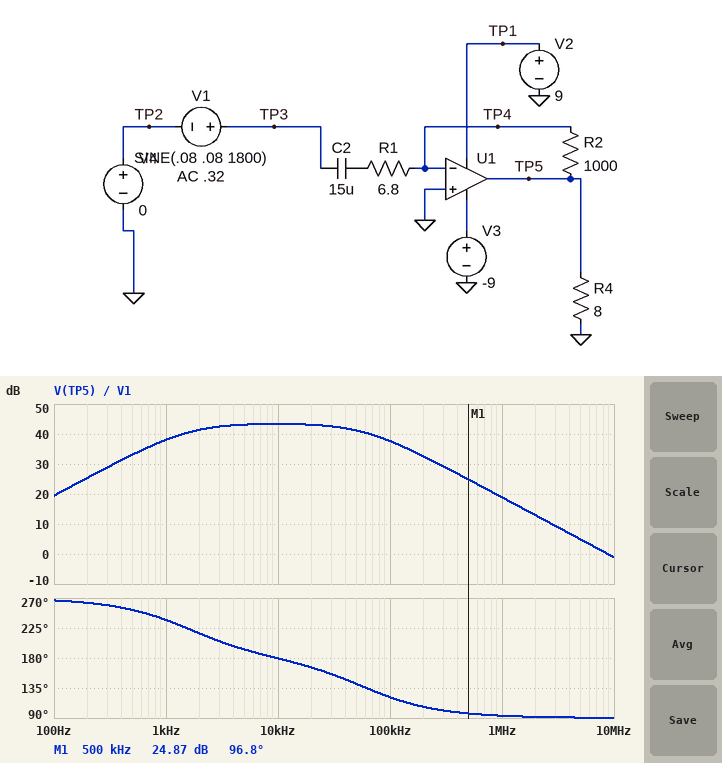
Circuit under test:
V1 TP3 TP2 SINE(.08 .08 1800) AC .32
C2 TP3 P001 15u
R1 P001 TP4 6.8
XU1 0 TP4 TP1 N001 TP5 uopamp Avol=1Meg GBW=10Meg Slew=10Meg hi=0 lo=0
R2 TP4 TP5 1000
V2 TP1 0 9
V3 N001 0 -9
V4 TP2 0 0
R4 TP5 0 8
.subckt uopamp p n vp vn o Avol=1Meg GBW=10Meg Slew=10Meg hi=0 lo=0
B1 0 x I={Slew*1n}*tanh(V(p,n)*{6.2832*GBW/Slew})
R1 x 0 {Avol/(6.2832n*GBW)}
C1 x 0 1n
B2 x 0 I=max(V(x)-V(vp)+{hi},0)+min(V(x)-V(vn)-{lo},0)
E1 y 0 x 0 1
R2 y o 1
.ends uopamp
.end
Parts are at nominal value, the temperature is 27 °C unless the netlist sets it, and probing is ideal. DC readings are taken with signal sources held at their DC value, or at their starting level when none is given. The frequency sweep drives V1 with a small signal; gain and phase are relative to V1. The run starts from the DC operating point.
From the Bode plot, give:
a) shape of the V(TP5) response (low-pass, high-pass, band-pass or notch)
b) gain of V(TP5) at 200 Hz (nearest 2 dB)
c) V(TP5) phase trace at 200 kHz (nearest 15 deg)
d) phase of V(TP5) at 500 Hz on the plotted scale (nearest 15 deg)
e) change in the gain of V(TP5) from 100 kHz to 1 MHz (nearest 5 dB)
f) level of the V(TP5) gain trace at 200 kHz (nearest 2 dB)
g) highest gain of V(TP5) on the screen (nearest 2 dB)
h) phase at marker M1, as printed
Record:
band-pass
26 dB
105 deg
255 deg
-20 dB
32 dB
44 dB
96.8 deg
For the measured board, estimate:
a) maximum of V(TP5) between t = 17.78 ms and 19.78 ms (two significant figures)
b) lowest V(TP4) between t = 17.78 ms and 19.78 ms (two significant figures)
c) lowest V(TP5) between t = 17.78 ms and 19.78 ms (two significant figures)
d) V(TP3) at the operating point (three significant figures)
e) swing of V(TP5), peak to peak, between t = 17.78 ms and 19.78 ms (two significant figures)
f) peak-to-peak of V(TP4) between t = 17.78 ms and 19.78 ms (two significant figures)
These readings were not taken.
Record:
8.0 V
-8.5 mV
-8.0 V
80.0 mV
16 V
17 mV
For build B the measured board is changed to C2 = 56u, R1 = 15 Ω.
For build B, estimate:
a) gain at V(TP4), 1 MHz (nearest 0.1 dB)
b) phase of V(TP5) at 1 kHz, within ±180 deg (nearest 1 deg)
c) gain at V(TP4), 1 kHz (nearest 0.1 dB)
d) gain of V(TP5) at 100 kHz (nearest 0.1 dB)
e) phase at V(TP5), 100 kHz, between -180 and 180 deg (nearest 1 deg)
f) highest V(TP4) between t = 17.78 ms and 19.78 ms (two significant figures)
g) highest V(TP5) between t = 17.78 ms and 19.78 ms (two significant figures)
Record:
-0.2 dB
-170 deg
-42.6 dB
34.5 dB
143 deg
1.1 mV
5.3 V
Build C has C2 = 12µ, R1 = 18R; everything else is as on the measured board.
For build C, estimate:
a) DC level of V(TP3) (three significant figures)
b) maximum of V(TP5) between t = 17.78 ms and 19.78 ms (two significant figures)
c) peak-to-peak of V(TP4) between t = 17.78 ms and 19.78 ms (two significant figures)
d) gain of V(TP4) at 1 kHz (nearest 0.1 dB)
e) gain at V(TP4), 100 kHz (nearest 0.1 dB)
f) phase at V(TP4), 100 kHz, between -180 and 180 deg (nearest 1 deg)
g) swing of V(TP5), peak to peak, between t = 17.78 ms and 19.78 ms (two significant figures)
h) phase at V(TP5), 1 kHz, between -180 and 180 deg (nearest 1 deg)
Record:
80.0 mV
4.1 V
1.7 mV
-45.9 dB
-5.5 dB
58 deg
8.3 V
-144 deg
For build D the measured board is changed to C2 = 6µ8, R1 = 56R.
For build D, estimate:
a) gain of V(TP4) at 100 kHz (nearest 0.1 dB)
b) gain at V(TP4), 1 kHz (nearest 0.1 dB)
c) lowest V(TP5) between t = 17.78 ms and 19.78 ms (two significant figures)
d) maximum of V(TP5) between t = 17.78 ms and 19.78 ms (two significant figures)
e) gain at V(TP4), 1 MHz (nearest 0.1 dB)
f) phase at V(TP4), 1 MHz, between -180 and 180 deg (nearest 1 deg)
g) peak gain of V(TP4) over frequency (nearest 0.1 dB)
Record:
-14.1 dB
-54.6 dB
-1.4 V
1.4 V
-1.3 dB
25 deg
-0.5 dB
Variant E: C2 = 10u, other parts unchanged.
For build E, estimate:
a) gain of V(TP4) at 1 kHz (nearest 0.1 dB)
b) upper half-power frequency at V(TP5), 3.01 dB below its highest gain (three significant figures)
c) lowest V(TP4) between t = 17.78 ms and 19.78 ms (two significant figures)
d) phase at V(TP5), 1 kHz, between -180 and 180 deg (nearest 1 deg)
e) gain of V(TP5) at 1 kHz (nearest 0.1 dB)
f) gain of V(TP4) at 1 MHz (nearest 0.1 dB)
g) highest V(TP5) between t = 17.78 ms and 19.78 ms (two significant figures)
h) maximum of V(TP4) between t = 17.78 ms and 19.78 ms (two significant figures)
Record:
-43.7 dB
62.3 kHz
-1.5 mV
-113 deg
35.3 dB
-0.1 dB
7.3 V
1.5 mV
